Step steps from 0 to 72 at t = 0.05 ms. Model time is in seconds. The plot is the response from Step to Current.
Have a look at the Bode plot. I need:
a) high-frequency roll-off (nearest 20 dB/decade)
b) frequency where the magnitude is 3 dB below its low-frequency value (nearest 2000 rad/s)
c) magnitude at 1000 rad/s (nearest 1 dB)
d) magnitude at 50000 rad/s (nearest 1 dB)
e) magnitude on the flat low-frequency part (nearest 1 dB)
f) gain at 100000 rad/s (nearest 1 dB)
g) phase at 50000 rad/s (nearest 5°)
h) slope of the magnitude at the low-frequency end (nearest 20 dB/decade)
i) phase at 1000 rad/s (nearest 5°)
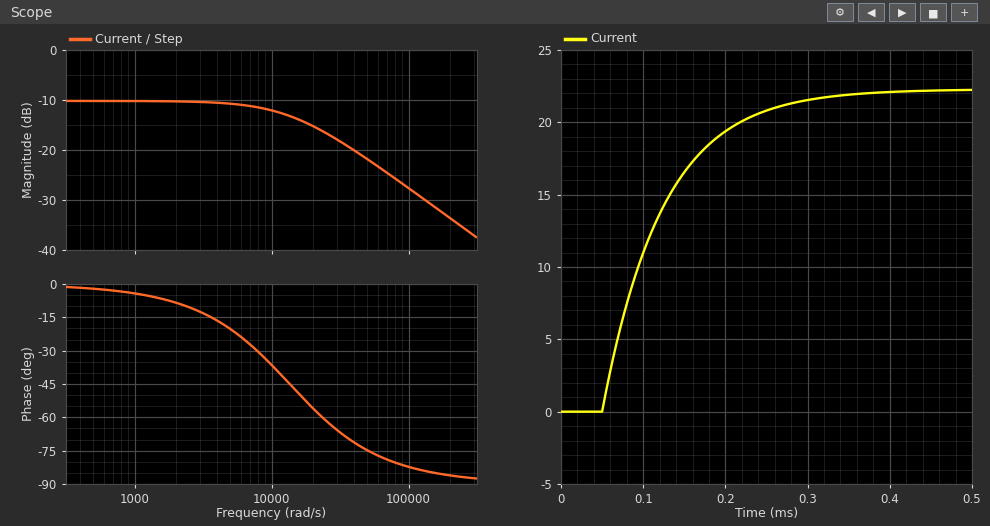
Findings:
-20 dB/decade
14000 rad/s
-10 dB
-22 dB
-10 dB
-28 dB
-75°
0 dB/decade
-5°
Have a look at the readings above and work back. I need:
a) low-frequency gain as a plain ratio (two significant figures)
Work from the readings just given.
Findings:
0.32
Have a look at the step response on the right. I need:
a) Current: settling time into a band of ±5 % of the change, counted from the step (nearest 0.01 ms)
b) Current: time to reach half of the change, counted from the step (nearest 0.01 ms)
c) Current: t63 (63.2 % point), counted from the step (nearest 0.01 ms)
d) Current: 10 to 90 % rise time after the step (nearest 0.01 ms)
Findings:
0.22 ms
0.05 ms
0.07 ms
0.16 ms
